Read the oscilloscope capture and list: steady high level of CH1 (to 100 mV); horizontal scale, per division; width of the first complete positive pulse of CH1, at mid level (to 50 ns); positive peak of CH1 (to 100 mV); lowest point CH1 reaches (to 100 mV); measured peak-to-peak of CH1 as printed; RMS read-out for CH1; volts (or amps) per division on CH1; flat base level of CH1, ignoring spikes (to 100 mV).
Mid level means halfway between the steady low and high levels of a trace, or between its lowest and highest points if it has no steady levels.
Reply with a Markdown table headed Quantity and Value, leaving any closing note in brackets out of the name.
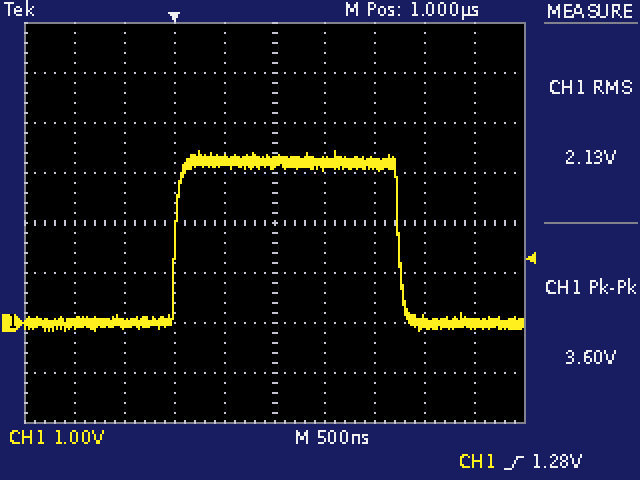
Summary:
| Quantity | Value |
|---|---|
| steady high level of CH1 | 3.2 V |
| horizontal scale, per division | 500 ns |
| width of the first complete positive pulse of CH1, at mid level | 2.25 µs |
| positive peak of CH1 | 3.4 V |
| lowest point CH1 reaches | -200 mV |
| measured peak-to-peak of CH1 as printed | 3.60 V |
| RMS read-out for CH1 | 2.13 V |
| volts (or amps) per division on CH1 | 1 V |
| flat base level of CH1, ignoring spikes | 0.0 V |
